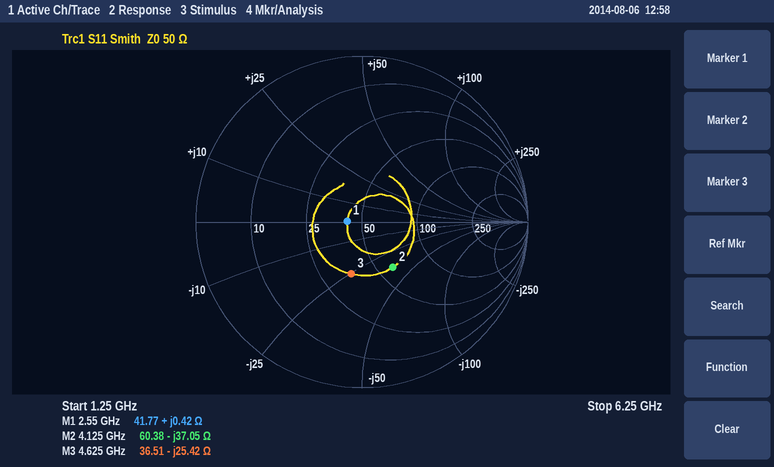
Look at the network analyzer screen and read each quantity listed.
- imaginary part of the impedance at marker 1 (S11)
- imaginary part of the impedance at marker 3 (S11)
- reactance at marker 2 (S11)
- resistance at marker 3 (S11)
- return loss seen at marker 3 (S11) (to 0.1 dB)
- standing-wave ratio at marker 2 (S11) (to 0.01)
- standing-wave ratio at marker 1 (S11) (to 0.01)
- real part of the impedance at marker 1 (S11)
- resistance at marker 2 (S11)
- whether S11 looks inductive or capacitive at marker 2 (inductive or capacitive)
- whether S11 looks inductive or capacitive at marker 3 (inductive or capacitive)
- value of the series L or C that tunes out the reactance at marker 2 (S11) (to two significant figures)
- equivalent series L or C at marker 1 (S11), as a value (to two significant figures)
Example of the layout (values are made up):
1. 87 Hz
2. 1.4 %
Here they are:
1. +0.42 Ω
2. -25.42 Ω
3. -37.05 Ω
4. 36.51 Ω
5. 9.9 dB
6. 1.99
7. 1.20
8. 41.77 Ω
9. 60.38 Ω
10. capacitive
11. capacitive
12. 1.4 nH
13. 26 pH
